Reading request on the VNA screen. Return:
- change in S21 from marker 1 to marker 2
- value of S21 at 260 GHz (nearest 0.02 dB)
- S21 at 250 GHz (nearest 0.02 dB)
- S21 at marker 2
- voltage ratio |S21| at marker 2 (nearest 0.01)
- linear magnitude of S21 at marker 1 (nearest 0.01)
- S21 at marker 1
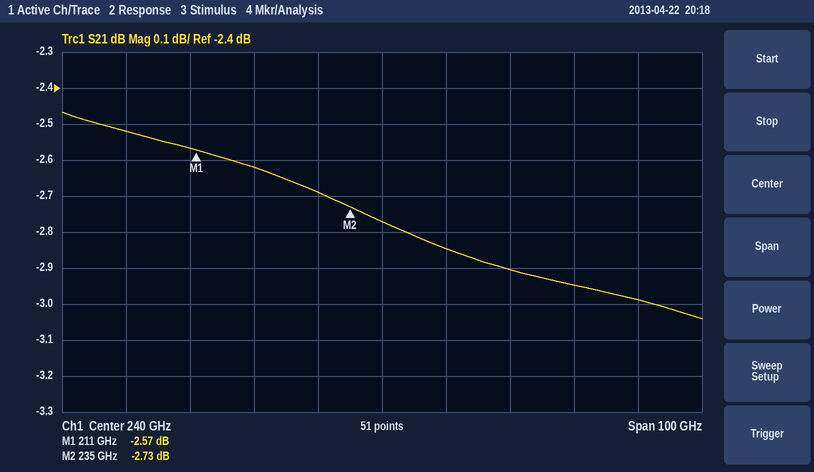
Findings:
-0.16 dB
-2.90 dB
-2.84 dB
-2.73 dB
0.73
0.74
-2.57 dB
